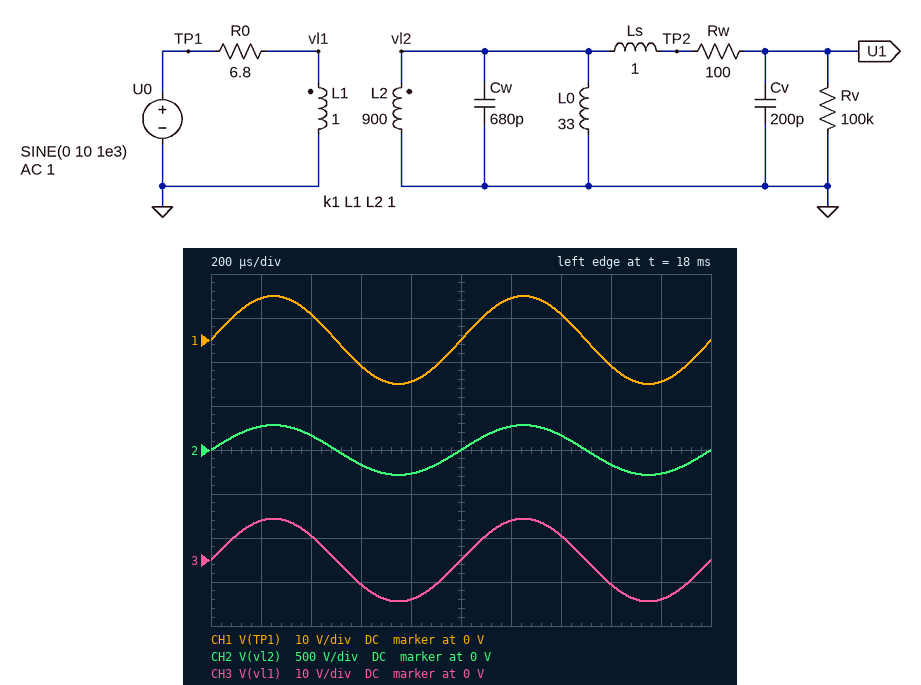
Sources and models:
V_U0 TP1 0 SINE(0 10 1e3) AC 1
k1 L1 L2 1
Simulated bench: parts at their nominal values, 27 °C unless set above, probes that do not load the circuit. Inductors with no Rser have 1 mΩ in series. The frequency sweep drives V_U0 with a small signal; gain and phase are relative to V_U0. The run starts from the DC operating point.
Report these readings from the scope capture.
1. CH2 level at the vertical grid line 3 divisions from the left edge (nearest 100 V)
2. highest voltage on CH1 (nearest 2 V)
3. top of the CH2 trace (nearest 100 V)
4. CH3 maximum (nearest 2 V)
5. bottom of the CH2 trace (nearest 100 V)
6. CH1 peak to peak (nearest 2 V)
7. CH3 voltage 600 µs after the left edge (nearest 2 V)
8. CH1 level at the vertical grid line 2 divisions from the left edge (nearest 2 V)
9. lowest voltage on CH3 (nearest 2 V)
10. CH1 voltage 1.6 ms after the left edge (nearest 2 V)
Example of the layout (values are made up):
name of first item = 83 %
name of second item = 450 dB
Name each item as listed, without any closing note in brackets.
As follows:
CH2 level at the vertical grid line 3 divisions from the left edge = -200 V
highest voltage on CH1 = 10 V
top of the CH2 trace = 300 V
CH3 maximum = 10 V
bottom of the CH2 trace = -300 V
CH1 peak to peak = 20 V
CH3 voltage 600 µs after the left edge = -6 V
CH1 level at the vertical grid line 2 divisions from the left edge = 6 V
lowest voltage on CH3 = -10 V
CH1 voltage 1.6 ms after the left edge = -6 V
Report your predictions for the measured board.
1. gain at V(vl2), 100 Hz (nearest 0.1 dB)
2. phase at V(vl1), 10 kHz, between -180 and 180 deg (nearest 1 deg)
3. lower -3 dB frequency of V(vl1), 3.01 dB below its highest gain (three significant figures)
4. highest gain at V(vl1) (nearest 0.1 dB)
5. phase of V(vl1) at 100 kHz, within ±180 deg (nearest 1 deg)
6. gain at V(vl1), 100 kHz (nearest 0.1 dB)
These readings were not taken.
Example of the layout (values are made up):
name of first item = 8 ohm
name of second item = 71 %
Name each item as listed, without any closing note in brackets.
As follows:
gain at V(vl2), 100 Hz = 28.7 dB
phase at V(vl1), 10 kHz, between -180 and 180 deg = -10 deg
lower -3 dB frequency of V(vl1), 3.01 dB below its highest gain = 28.8 Hz
highest gain at V(vl1) = -0.5 dB
phase of V(vl1) at 100 kHz, within ±180 deg = -69 deg
gain at V(vl1), 100 kHz = -8.9 dB
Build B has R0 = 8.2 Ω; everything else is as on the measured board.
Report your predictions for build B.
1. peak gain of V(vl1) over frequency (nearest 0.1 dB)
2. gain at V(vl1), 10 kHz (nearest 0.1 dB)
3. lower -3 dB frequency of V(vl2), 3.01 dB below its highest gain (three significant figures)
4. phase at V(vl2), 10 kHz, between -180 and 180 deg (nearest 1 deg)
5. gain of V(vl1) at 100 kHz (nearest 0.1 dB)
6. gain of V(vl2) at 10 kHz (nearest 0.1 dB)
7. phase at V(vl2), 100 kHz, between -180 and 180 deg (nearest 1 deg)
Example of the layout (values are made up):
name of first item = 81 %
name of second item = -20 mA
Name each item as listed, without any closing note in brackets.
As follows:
peak gain of V(vl1) over frequency = -0.6 dB
gain at V(vl1), 10 kHz = -1.5 dB
lower -3 dB frequency of V(vl2), 3.01 dB below its highest gain = 34.3 Hz
phase at V(vl2), 10 kHz, between -180 and 180 deg = -12 deg
gain of V(vl1) at 100 kHz = -10.4 dB
gain of V(vl2) at 10 kHz = 28.0 dB
phase at V(vl2), 100 kHz, between -180 and 180 deg = -72 deg
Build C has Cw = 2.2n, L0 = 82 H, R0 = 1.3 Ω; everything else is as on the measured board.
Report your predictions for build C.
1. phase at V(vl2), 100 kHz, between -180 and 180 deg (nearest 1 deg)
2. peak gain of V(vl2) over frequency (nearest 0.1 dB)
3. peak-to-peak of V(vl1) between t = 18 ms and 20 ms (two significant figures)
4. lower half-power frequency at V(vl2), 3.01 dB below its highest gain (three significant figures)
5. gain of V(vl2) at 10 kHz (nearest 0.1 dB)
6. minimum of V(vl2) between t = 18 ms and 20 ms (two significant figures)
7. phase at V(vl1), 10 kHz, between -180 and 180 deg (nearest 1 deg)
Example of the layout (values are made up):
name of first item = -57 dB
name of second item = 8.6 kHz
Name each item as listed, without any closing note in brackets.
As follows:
phase at V(vl2), 100 kHz, between -180 and 180 deg = -58 deg
peak gain of V(vl2) over frequency = 29.4 dB
peak-to-peak of V(vl1) between t = 18 ms and 20 ms = 20 V
lower half-power frequency at V(vl2), 3.01 dB below its highest gain = 2.45 Hz
gain of V(vl2) at 10 kHz = 29.2 dB
minimum of V(vl2) between t = 18 ms and 20 ms = -300 V
phase at V(vl1), 10 kHz, between -180 and 180 deg = -8 deg
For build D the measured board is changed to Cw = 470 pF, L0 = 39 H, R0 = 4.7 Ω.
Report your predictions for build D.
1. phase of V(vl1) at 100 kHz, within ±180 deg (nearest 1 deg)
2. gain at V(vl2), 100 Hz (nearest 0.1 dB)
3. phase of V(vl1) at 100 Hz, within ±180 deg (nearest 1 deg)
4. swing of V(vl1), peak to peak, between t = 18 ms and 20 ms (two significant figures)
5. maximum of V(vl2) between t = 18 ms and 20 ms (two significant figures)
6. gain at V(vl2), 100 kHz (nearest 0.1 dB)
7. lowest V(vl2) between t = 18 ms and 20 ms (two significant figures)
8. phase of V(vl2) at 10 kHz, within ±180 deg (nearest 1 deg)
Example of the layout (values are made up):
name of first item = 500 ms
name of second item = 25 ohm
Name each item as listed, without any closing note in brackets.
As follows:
phase of V(vl1) at 100 kHz, within ±180 deg = -51 deg
gain at V(vl2), 100 Hz = 29.1 dB
phase of V(vl1) at 100 Hz, within ±180 deg = 10 deg
swing of V(vl1), peak to peak, between t = 18 ms and 20 ms = 19 V
maximum of V(vl2) between t = 18 ms and 20 ms = 290 V
gain at V(vl2), 100 kHz = 25.5 dB
lowest V(vl2) between t = 18 ms and 20 ms = -290 V
phase of V(vl2) at 10 kHz, within ±180 deg = -5 deg
